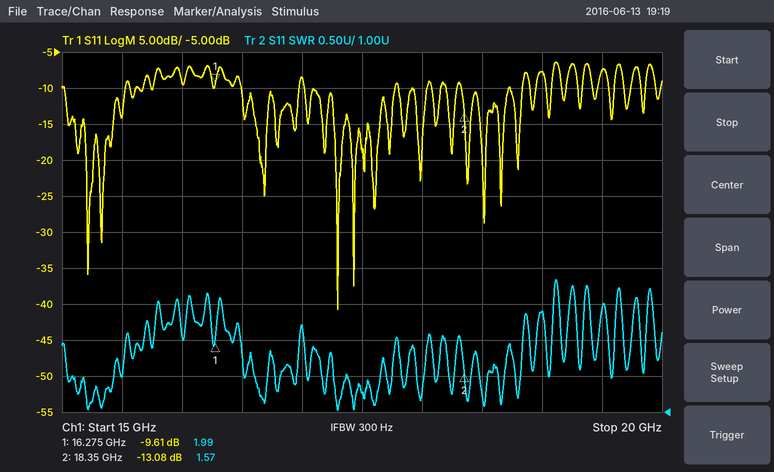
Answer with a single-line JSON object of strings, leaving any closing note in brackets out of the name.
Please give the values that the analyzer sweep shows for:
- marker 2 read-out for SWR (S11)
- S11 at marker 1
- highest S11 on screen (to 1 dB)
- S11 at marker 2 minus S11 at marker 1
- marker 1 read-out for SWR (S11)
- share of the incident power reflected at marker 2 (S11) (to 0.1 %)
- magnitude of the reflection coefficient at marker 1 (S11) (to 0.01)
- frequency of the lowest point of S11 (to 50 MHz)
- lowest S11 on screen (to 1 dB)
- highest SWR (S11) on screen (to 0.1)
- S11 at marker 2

{"marker 2 read-out for SWR": "1.57", "S11 at marker 1": "-9.61 dB", "highest S11 on screen": "-6 dB", "S11 at marker 2 minus S11 at marker 1": "-3.47 dB", "marker 1 read-out for SWR": "1.99", "share of the incident power reflected at marker 2 (S11)": "4.9 %", "magnitude of the reflection coefficient at marker 1 (S11)": "0.33", "frequency of the lowest point of S11": "17.30 GHz", "lowest S11 on screen": "-41 dB", "highest SWR (S11) on screen": "2.8", "S11 at marker 2": "-13.08 dB"}
